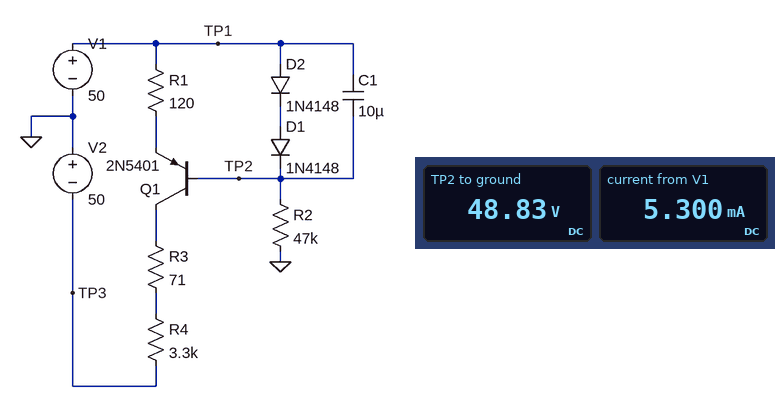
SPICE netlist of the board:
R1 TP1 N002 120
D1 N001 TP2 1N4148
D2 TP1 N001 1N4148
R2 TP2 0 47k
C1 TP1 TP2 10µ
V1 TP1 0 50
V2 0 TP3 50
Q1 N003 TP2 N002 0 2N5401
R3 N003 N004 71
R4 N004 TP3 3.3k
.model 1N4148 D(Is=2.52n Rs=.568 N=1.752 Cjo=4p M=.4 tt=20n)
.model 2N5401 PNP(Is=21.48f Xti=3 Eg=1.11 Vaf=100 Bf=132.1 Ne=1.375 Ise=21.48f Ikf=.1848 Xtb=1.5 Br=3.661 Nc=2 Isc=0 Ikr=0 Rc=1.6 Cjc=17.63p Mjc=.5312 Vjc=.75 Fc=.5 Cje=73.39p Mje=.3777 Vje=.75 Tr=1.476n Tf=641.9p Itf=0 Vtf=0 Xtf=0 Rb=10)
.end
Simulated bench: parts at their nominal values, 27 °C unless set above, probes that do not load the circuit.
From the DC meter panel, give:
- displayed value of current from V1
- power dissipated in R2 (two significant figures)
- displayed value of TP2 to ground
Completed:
5.300 mA
51 mW
48.83 V
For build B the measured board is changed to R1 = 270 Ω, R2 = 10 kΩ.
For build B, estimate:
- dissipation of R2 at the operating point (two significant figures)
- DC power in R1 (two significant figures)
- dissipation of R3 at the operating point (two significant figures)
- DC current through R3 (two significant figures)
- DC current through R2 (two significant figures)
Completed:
240 mW
1.7 mW
440 µW
2.5 mA
4.9 mA
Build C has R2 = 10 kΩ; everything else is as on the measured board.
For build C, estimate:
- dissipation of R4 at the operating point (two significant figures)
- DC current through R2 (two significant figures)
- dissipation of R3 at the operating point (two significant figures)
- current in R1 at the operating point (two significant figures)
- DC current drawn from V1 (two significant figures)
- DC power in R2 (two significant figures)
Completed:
97 mW
4.9 mA
2.1 mW
5.4 mA
10 mA
240 mW
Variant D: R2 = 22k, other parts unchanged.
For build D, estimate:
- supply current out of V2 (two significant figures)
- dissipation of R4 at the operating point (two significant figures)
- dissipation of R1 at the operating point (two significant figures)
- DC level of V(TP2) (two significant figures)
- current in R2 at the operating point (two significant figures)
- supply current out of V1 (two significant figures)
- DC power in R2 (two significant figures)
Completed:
4.8 mA
77 mW
2.8 mW
49 V
2.2 mA
7.0 mA
110 mW
